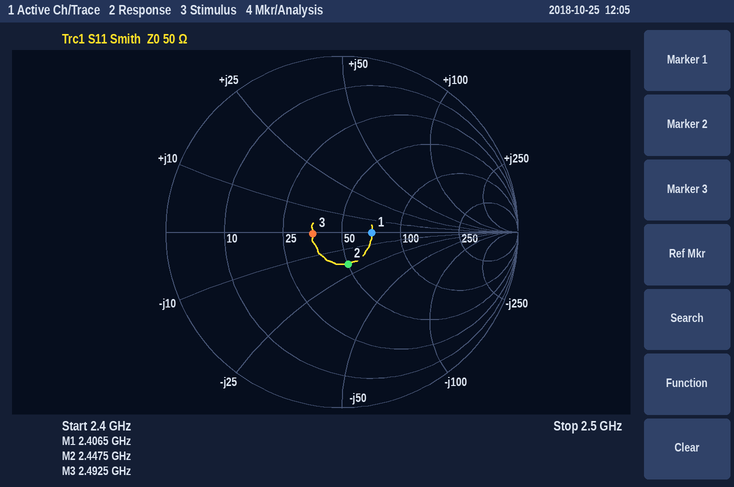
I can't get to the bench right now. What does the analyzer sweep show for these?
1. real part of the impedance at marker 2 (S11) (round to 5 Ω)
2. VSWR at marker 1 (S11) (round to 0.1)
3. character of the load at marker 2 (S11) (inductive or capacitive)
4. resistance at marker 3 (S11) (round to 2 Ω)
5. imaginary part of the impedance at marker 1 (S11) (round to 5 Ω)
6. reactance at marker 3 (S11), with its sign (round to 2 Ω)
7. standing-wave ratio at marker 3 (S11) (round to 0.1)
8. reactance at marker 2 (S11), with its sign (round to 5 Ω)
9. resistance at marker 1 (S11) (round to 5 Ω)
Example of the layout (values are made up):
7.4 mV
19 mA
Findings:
50 Ω
1.4
capacitive
36 Ω
0 Ω
0 Ω
1.4
-20 Ω
70 Ω
